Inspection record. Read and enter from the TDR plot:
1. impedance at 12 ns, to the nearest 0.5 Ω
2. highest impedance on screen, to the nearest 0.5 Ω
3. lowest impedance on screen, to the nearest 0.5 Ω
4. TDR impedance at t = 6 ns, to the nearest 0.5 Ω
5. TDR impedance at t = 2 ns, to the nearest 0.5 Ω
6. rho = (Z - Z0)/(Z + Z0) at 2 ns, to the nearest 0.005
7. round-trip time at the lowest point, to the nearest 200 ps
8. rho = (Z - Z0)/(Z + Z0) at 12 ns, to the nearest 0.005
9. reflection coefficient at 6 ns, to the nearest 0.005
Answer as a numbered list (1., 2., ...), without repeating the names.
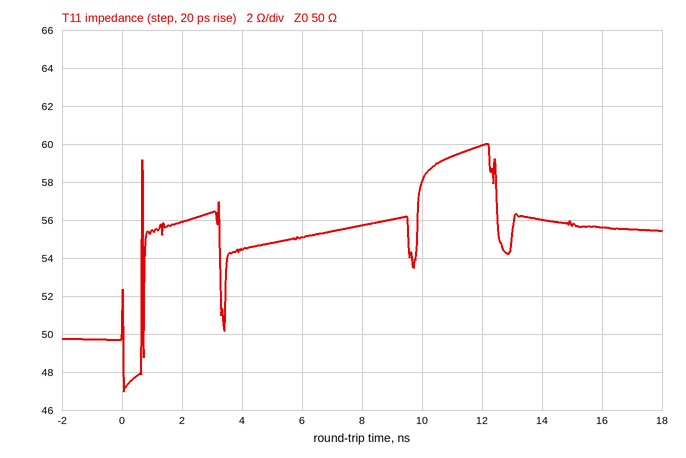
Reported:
1. 60.0 Ω
2. 60.0 Ω
3. 47.0 Ω
4. 55.0 Ω
5. 56.0 Ω
6. +0.055
7. 0.0 ns
8. +0.090
9. +0.050
